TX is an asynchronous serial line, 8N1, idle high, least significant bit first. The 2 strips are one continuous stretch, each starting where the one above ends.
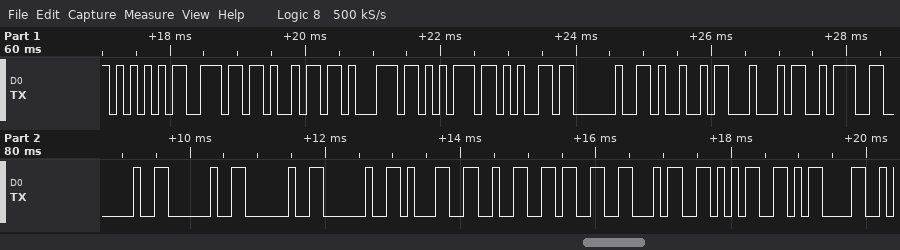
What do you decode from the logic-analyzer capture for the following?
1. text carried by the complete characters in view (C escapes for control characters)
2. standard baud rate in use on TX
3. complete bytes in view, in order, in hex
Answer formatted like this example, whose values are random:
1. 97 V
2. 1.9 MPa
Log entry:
1. "Unique ID:    12345\r"
2. 9600 baud
3. 55 6E 69 71 75 65 20 49 44 3A 20 20 20 20 31 32 33 34 35 0D
